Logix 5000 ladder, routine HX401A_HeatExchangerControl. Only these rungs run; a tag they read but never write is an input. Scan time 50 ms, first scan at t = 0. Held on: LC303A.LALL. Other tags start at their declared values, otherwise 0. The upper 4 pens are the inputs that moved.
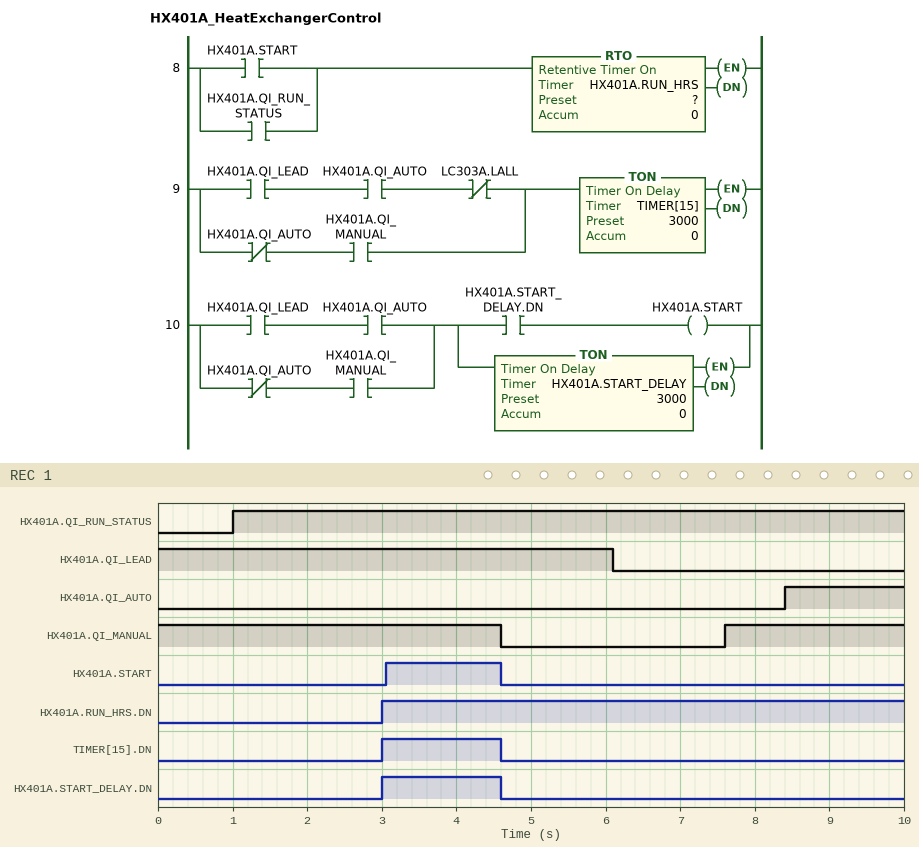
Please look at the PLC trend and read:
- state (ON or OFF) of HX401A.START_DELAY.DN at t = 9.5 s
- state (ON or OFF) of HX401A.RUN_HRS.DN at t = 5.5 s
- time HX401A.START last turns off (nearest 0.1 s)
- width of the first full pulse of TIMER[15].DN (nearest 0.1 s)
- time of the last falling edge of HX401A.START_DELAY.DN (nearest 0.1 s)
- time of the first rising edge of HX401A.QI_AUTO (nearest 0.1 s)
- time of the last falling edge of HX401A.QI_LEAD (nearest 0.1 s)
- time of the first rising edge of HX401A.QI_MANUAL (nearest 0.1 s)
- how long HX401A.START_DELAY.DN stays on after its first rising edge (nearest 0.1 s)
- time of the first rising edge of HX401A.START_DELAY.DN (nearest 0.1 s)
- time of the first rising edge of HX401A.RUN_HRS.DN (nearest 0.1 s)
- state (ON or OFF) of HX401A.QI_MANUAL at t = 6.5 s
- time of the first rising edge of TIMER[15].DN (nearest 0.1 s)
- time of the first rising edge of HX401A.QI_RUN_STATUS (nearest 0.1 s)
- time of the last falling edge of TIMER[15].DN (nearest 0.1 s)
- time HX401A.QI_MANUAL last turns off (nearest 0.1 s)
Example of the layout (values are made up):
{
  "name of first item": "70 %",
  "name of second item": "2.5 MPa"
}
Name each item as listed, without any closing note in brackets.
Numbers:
{
  "state (ON or OFF) of HX401A.START_DELAY.DN at t = 9.5 s": "OFF",
  "state (ON or OFF) of HX401A.RUN_HRS.DN at t = 5.5 s": "ON",
  "time HX401A.START last turns off": "4.6 s",
  "width of the first full pulse of TIMER[15].DN": "1.6 s",
  "time of the last falling edge of HX401A.START_DELAY.DN": "4.6 s",
  "time of the first rising edge of HX401A.QI_AUTO": "8.4 s",
  "time of the last falling edge of HX401A.QI_LEAD": "6.1 s",
  "time of the first rising edge of HX401A.QI_MANUAL": "7.6 s",
  "how long HX401A.START_DELAY.DN stays on after its first rising edge": "1.6 s",
  "time of the first rising edge of HX401A.START_DELAY.DN": "3.0 s",
  "time of the first rising edge of HX401A.RUN_HRS.DN": "3.0 s",
  "state (ON or OFF) of HX401A.QI_MANUAL at t = 6.5 s": "OFF",
  "time of the first rising edge of TIMER[15].DN": "3.0 s",
  "time of the first rising edge of HX401A.QI_RUN_STATUS": "1.0 s",
  "time of the last falling edge of TIMER[15].DN": "4.6 s",
  "time HX401A.QI_MANUAL last turns off": "4.6 s"
}
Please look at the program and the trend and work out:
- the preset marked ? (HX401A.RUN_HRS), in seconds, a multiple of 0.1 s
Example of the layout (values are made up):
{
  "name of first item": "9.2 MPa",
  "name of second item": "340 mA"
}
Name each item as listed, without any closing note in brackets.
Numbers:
{
  "the preset marked ? (HX401A.RUN_HRS), in seconds, a multiple of 0.1 s": "2.0 s"
}
